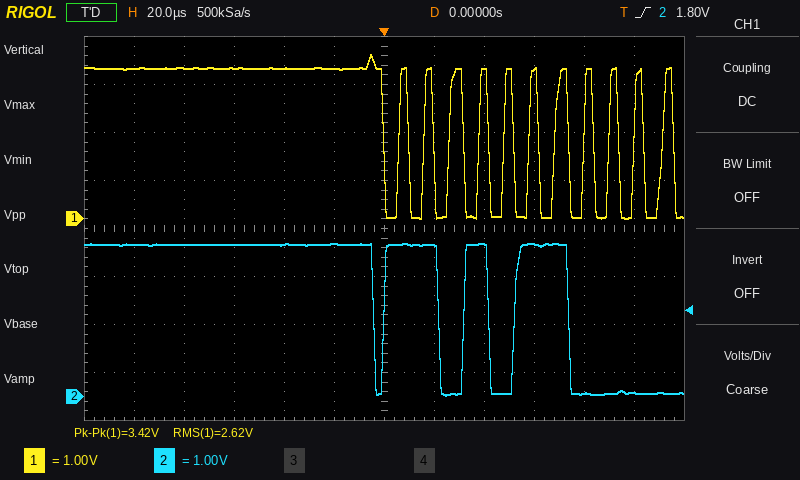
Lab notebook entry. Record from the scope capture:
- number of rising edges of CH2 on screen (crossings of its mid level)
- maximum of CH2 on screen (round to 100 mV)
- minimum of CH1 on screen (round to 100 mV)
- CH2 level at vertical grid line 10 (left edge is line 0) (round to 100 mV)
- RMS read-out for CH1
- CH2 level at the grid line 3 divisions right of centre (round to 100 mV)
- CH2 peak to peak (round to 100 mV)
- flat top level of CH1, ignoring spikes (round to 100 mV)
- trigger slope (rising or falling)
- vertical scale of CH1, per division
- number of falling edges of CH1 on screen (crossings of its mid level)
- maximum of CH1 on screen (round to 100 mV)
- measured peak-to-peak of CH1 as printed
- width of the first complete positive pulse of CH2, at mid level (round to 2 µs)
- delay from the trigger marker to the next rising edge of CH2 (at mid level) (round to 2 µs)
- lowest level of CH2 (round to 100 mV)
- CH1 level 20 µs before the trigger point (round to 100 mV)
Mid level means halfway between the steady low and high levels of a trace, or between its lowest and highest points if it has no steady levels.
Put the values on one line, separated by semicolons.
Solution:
3; 3.2 V; 0.0 V; 100 mV; 2.62 V; 3.2 V; 3.2 V; 3.1 V; rising; 1 V; 12; 3.4 V; 3.42 V; 22 µs; 32 µs; 0.0 V; 3.1 V
